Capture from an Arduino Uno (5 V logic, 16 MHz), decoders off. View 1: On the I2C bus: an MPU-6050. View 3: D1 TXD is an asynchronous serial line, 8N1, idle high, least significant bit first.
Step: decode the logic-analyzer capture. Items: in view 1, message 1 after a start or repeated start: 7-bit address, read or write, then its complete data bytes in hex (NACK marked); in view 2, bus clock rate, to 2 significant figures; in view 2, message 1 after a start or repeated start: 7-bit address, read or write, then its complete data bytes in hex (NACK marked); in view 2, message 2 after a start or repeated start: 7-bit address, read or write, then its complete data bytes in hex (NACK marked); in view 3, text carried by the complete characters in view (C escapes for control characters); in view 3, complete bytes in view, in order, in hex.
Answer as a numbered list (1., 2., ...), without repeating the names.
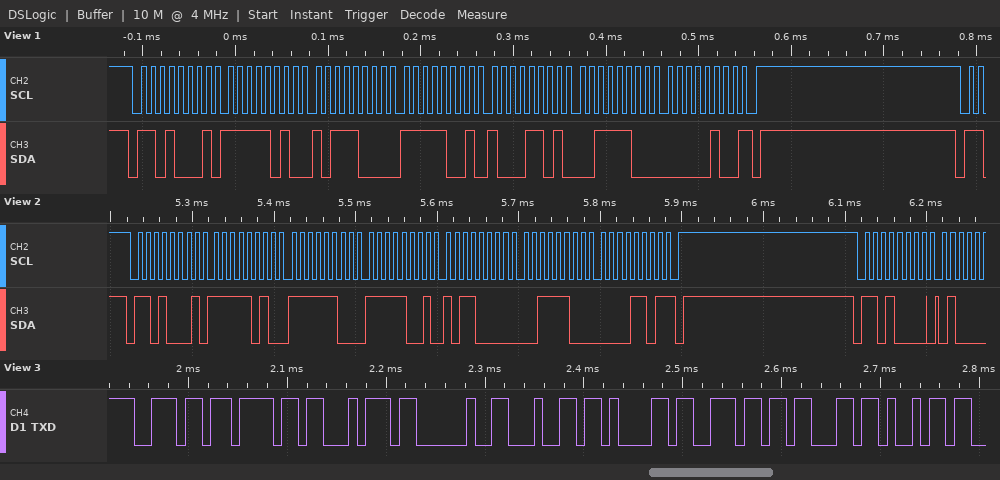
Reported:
1. 0x68 read: FA B8 F9 8D 3C 04 NACK
2. 100 kHz
3. 0x68 read: FA FC F9 B0 3C 0D NACK
4. 0x68 write
5. "not danci"
6. 6E 6F 74 20 64 61 6E 63 69
